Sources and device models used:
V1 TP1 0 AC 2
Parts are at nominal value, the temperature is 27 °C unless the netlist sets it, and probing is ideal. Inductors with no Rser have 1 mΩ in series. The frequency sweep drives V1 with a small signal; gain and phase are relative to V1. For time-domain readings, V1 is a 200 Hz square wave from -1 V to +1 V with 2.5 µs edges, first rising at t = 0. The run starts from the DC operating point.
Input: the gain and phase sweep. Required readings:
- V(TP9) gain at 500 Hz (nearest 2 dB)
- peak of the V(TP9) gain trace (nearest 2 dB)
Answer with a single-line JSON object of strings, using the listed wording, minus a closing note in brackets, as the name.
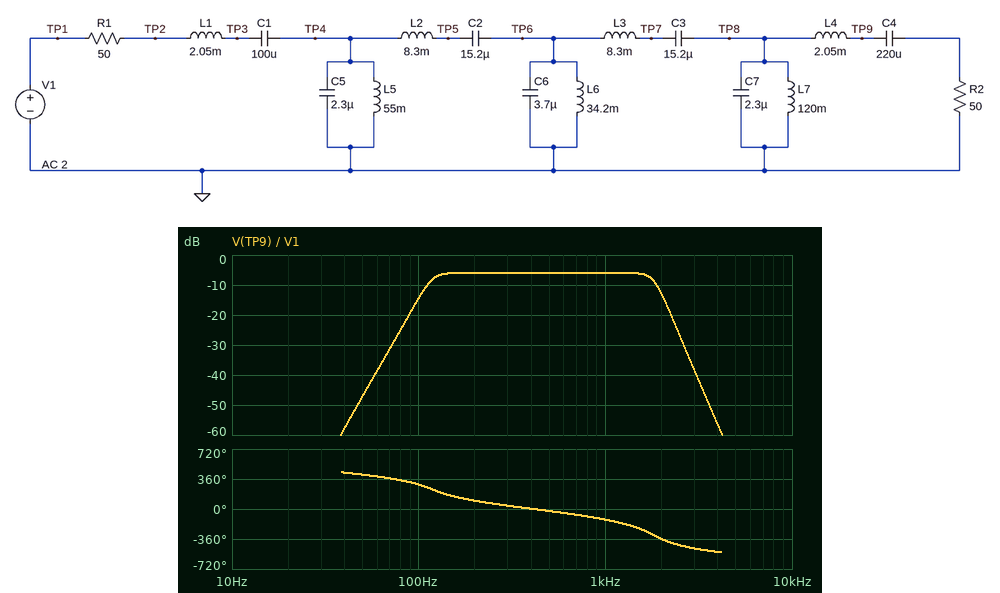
{"V(TP9) gain at 500 Hz": "-6 dB", "peak of the V(TP9) gain trace": "-6 dB"}
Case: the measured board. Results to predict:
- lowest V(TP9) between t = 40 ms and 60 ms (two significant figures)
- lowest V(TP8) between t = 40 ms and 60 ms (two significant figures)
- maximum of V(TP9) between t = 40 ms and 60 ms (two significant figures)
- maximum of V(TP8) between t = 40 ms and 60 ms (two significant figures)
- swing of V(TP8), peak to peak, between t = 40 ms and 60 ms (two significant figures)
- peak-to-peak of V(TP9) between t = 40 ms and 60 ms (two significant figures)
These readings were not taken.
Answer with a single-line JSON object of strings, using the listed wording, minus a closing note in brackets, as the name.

{"lowest V(TP9) between t = 40 ms and 60 ms": "-880 mV", "lowest V(TP8) between t = 40 ms and 60 ms": "-900 mV", "maximum of V(TP9) between t = 40 ms and 60 ms": "880 mV", "maximum of V(TP8) between t = 40 ms and 60 ms": "900 mV", "swing of V(TP8), peak to peak, between t = 40 ms and 60 ms": "1.8 V", "peak-to-peak of V(TP9) between t = 40 ms and 60 ms": "1.8 V"}
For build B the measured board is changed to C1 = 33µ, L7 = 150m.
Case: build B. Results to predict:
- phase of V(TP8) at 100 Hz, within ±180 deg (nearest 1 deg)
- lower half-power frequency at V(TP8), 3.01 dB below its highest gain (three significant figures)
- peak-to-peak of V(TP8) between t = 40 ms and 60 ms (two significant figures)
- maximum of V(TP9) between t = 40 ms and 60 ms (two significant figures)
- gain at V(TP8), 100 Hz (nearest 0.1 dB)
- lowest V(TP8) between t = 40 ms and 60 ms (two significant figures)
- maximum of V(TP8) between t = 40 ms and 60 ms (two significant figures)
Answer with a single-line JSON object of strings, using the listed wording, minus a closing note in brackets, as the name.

{"phase of V(TP8) at 100 Hz, within ±180 deg": "-50 deg", "lower half-power frequency at V(TP8), 3.01 dB below its highest gain": "115 Hz", "peak-to-peak of V(TP8) between t = 40 ms and 60 ms": "1.7 V", "maximum of V(TP9) between t = 40 ms and 60 ms": "820 mV", "gain at V(TP8), 100 Hz": "-12.3 dB", "lowest V(TP8) between t = 40 ms and 60 ms": "-830 mV", "maximum of V(TP8) between t = 40 ms and 60 ms": "830 mV"}
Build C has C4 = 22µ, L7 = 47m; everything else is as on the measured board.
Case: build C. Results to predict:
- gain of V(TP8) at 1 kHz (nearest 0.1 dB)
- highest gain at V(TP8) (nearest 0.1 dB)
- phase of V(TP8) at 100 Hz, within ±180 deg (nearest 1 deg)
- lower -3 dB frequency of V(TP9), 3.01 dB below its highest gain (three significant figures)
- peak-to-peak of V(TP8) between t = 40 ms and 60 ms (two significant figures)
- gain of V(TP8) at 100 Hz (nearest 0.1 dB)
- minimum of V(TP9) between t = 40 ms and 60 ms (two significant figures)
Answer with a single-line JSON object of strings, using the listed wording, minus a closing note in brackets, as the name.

{"gain of V(TP8) at 1 kHz": "-6.0 dB", "highest gain at V(TP8)": "-2.5 dB", "phase of V(TP8) at 100 Hz, within ±180 deg": "-2 deg", "lower -3 dB frequency of V(TP9), 3.01 dB below its highest gain": "104 Hz", "peak-to-peak of V(TP8) between t = 40 ms and 60 ms": "1.9 V", "gain of V(TP8) at 100 Hz": "-8.9 dB", "minimum of V(TP9) between t = 40 ms and 60 ms": "-970 mV"}
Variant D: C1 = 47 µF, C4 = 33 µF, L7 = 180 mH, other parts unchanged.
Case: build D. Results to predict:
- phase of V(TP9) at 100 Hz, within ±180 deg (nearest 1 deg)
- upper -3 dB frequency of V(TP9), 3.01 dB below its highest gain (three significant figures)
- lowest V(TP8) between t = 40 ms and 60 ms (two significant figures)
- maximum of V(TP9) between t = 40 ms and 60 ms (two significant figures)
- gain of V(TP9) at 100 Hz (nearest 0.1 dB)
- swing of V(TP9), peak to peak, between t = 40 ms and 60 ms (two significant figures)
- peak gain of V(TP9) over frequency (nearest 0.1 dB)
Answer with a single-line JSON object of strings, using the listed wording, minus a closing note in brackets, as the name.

{"phase of V(TP9) at 100 Hz, within ±180 deg": "-97 deg", "upper -3 dB frequency of V(TP9), 3.01 dB below its highest gain": "1.81 kHz", "lowest V(TP8) between t = 40 ms and 60 ms": "-970 mV", "maximum of V(TP9) between t = 40 ms and 60 ms": "970 mV", "gain of V(TP9) at 100 Hz": "-12.6 dB", "swing of V(TP9), peak to peak, between t = 40 ms and 60 ms": "1.9 V", "peak gain of V(TP9) over frequency": "-5.6 dB"}
